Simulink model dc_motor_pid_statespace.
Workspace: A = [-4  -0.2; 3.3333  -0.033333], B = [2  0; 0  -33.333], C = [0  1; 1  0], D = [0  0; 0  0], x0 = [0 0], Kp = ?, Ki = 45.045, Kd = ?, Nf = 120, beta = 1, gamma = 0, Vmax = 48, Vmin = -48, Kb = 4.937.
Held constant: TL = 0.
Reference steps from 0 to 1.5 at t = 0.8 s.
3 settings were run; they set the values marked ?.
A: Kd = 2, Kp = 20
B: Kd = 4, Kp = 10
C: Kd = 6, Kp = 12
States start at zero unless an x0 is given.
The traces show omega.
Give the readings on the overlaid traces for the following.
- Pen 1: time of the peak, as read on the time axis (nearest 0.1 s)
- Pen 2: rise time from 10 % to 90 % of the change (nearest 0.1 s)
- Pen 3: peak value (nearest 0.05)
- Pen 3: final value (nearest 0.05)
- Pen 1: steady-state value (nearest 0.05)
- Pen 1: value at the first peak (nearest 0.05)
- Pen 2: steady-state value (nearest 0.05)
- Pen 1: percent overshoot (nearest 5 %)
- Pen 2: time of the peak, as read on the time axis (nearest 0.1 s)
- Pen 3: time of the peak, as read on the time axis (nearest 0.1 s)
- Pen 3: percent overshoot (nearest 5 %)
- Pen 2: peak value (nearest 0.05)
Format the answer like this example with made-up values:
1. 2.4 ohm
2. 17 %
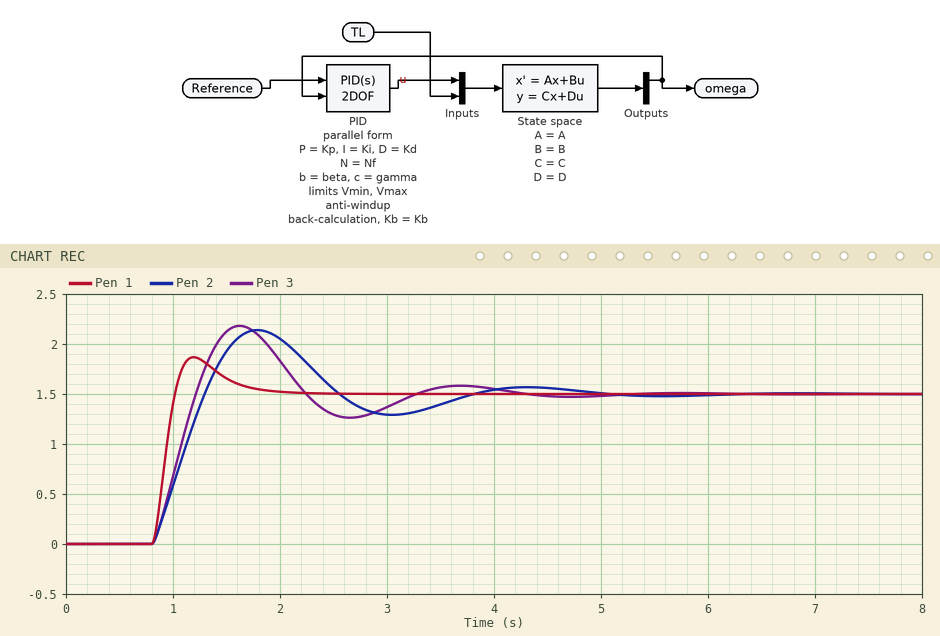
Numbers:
1. 1.2 s
2. 0.4 s
3. 2.20
4. 1.50
5. 1.50
6. 1.85
7. 1.50
8. 25 %
9. 1.8 s
10. 1.6 s
11. 45 %
12. 2.15
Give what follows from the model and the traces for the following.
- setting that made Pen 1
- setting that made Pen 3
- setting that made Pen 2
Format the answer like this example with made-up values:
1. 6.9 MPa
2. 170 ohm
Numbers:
1. A
2. B
3. C
